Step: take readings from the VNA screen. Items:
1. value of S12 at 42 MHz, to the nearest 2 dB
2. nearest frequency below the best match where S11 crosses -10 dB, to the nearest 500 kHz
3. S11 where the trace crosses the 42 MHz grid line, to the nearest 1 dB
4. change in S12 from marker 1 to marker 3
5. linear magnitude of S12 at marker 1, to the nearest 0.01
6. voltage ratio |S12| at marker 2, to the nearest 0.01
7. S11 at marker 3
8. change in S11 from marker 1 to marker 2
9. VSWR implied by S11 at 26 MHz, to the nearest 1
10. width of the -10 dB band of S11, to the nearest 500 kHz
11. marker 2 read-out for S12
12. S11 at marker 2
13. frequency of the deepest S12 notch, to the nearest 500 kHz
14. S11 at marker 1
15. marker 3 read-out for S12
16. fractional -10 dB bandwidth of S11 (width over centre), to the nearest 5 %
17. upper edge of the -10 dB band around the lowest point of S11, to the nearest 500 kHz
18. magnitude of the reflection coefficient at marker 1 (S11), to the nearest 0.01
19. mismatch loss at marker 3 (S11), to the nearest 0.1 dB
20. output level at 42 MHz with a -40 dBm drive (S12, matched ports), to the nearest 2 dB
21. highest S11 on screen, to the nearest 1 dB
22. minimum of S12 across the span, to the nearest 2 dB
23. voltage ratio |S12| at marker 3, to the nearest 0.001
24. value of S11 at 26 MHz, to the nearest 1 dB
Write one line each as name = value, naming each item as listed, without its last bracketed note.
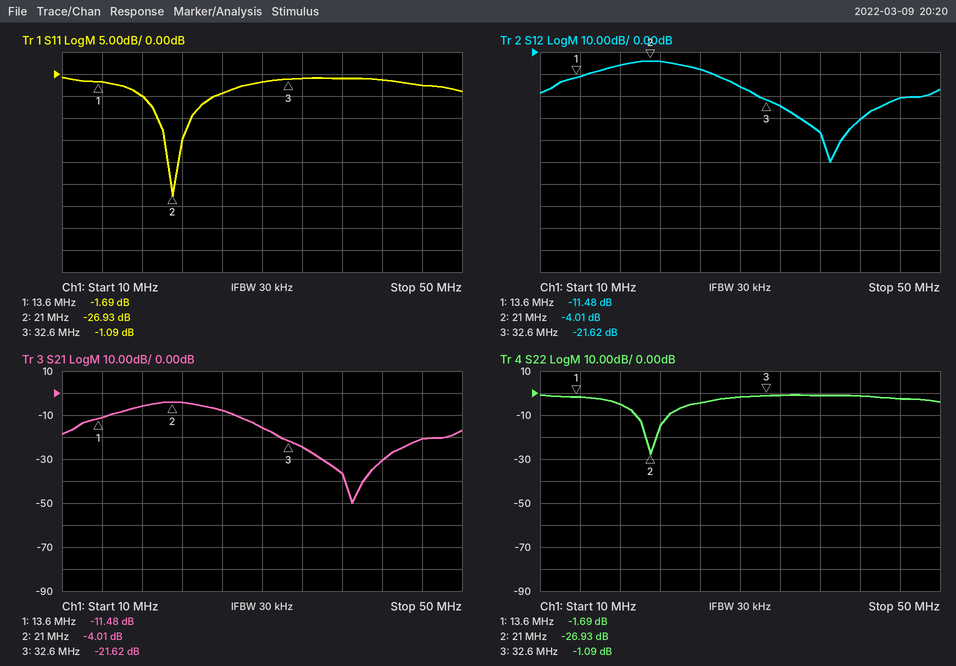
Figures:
value of S12 at 42 MHz, to the nearest 2 dB = -30 dB
nearest frequency below the best match where S11 crosses -10 dB, to the nearest 500 kHz = 19.5 MHz
S11 where the trace crosses the 42 MHz grid line, to the nearest 1 dB = -1 dB
change in S12 from marker 1 to marker 3 = -10.14 dB
linear magnitude of S12 at marker 1, to the nearest 0.01 = 0.27
voltage ratio |S12| at marker 2, to the nearest 0.01 = 0.63
S11 at marker 3 = -1.09 dB
change in S11 from marker 1 to marker 2 = -25.24 dB
VSWR implied by S11 at 26 MHz, to the nearest 1 = 4
width of the -10 dB band of S11, to the nearest 500 kHz = 3.5 MHz
marker 2 read-out for S12 = -4.01 dB
S11 at marker 2 = -26.93 dB
frequency of the deepest S12 notch, to the nearest 500 kHz = 39.0 MHz
S11 at marker 1 = -1.69 dB
marker 3 read-out for S12 = -21.62 dB
fractional -10 dB bandwidth of S11 (width over centre), to the nearest 5 % = 15 %
upper edge of the -10 dB band around the lowest point of S11, to the nearest 500 kHz = 23.0 MHz
magnitude of the reflection coefficient at marker 1 (S11), to the nearest 0.01 = 0.82
mismatch loss at marker 3 (S11), to the nearest 0.1 dB = 6.5 dB
output level at 42 MHz with a -40 dBm drive (S12, matched ports), to the nearest 2 dB = -70 dBm
highest S11 on screen, to the nearest 1 dB = -1 dB
minimum of S12 across the span, to the nearest 2 dB = -50 dB
voltage ratio |S12| at marker 3, to the nearest 0.001 = 0.083
value of S11 at 26 MHz, to the nearest 1 dB = -4 dB
